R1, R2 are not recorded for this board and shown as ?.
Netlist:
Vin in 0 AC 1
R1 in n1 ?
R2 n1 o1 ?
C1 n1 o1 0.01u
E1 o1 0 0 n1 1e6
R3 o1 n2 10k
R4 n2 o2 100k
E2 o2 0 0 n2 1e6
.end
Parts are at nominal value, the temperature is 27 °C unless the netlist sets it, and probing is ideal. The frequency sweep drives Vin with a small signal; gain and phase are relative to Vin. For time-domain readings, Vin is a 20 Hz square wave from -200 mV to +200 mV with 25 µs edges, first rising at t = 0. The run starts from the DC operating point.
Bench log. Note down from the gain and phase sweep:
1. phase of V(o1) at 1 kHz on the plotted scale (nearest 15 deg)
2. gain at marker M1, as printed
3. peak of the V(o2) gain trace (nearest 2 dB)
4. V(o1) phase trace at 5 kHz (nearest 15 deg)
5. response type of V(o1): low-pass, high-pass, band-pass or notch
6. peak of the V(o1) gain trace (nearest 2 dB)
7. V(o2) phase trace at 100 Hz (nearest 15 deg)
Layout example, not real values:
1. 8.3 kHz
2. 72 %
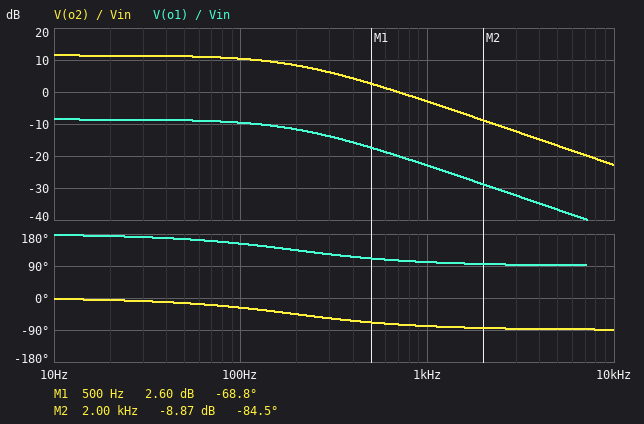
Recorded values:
1. 105 deg
2. 2.60 dB
3. 12 dB
4. 90 deg
5. low-pass
6. -8 dB
7. -30 deg
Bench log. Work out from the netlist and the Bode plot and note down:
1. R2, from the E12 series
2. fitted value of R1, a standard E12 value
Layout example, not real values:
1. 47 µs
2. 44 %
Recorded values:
1. 82 kΩ
2. 220 kΩ
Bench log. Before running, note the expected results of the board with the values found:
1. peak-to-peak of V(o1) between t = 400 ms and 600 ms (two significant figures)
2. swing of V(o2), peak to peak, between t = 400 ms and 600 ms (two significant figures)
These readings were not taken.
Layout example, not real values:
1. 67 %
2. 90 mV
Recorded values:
1. 150 mV
2. 1.5 V
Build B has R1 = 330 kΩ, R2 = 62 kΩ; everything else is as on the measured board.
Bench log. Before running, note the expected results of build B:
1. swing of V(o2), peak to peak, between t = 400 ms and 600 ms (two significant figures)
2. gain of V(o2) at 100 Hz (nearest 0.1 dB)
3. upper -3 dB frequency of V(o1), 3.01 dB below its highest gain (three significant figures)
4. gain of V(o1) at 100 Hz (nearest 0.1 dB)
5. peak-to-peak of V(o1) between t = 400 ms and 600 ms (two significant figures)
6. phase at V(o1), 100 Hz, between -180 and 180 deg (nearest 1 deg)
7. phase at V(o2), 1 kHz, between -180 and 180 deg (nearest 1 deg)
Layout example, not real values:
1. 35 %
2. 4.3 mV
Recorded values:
1. 750 mV
2. 4.9 dB
3. 257 Hz
4. -15.1 dB
5. 75 mV
6. 159 deg
7. -76 deg
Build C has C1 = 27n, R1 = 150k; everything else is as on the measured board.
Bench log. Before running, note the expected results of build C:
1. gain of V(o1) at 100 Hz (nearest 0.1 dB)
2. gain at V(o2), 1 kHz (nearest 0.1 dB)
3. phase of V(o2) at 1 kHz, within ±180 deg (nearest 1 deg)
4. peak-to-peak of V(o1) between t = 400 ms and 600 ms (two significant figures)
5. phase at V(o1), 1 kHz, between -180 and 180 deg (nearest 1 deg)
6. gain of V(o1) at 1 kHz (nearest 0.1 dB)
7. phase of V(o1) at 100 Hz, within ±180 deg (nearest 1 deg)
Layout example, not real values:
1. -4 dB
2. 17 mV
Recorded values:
1. -9.9 dB
2. -8.1 dB
3. -86 deg
4. 220 mV
5. 94 deg
6. -28.1 dB
7. 126 deg
